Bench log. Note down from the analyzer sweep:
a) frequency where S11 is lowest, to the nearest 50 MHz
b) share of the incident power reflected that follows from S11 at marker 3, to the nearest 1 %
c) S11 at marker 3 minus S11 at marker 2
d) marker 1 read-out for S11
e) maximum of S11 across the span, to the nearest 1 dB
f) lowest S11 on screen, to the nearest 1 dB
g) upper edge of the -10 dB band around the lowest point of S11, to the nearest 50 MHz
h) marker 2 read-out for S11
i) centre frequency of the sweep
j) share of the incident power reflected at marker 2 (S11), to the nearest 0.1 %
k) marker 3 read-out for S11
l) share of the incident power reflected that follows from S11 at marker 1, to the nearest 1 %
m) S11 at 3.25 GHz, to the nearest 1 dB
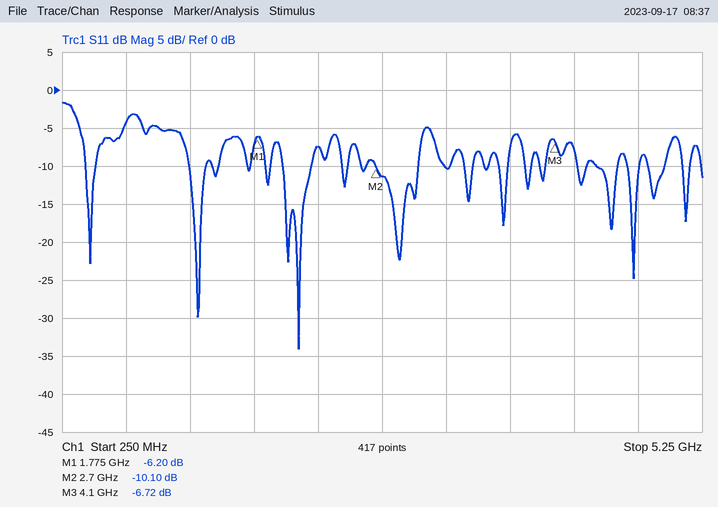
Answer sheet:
2.10 GHz
21 %
3.38 dB
-6.20 dB
-2 dB
-34 dB
2.20 GHz
-10.10 dB
2.75 GHz
9.8 %
-6.72 dB
24 %
-10 dB
